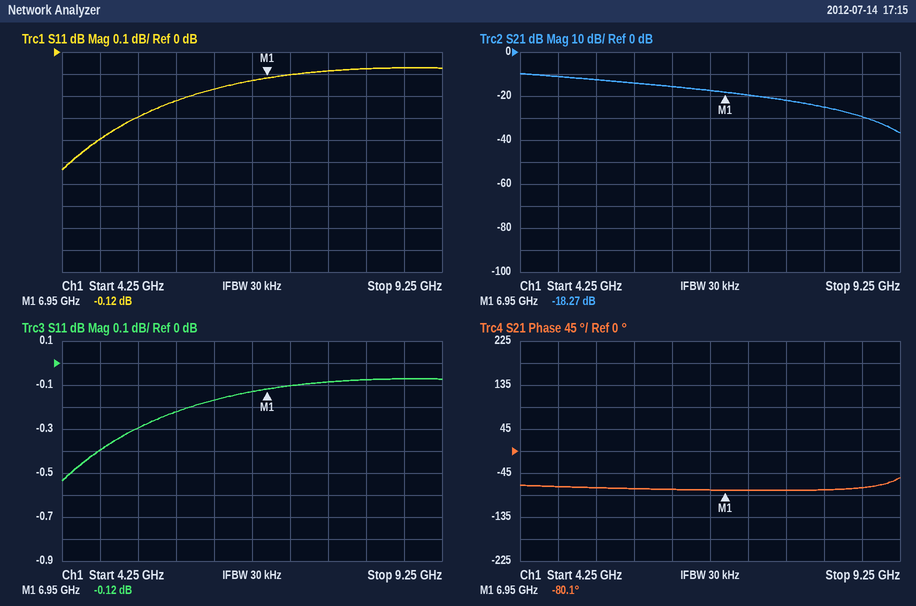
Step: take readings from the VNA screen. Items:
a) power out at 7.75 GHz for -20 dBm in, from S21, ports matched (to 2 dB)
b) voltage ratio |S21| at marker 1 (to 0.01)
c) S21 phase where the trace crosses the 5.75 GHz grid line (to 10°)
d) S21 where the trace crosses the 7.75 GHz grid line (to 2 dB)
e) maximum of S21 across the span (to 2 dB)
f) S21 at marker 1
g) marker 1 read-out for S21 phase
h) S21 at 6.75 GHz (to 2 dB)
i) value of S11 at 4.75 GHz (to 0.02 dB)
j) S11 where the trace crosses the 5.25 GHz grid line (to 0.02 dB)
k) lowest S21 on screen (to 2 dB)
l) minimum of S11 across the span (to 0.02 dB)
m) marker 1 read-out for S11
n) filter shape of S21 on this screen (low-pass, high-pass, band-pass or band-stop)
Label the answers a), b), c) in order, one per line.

a) -42 dBm
b) 0.12
c) -80°
d) -22 dB
e) -10 dB
f) -18.27 dB
g) -80.1°
h) -18 dB
i) -0.40 dB
j) -0.30 dB
k) -36 dB
l) -0.54 dB
m) -0.12 dB
n) low-pass
